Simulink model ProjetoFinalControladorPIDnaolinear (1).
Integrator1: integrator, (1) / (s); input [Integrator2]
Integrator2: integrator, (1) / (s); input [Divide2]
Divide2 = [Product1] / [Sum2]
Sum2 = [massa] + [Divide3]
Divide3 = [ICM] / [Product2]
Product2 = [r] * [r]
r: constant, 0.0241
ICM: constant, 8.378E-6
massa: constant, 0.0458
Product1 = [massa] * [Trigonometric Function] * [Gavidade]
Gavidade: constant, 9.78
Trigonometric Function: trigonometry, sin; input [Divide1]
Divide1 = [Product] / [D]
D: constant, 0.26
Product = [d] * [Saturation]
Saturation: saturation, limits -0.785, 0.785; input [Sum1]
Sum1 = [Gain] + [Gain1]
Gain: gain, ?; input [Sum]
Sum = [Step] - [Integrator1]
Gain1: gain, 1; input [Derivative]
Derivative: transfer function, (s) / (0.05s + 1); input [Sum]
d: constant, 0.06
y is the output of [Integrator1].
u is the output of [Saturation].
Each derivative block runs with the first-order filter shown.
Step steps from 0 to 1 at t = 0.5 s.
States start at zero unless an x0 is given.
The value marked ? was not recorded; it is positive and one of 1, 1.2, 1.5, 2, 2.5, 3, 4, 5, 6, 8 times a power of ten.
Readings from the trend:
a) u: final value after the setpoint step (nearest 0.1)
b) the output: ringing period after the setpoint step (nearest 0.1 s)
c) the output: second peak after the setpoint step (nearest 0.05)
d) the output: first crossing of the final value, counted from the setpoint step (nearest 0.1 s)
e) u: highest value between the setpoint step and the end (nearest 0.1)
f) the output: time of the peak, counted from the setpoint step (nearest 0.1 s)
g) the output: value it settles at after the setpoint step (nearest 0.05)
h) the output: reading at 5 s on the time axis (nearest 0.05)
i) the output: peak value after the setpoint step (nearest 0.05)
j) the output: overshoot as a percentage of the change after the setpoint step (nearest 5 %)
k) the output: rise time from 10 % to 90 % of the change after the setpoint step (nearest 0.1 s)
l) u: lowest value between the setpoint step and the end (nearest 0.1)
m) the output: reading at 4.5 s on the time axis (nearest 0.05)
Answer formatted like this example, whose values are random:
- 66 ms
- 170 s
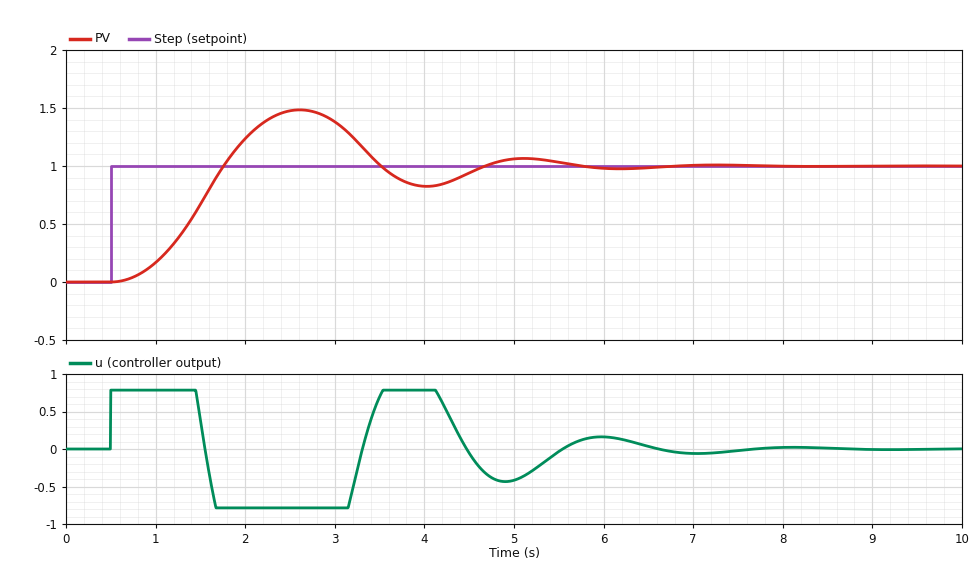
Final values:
- 0.0
- 2.5 s
- 1.05
- 1.3 s
- 0.8
- 2.1 s
- 1.00
- 1.05
- 1.50
- 50 %
- 0.8 s
- -0.8
- 0.95
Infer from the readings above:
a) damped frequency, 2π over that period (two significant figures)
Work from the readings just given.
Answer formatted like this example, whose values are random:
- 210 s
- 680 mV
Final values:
- 2.5 rad/s
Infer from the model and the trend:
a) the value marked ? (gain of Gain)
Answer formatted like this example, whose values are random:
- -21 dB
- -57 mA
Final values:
- 5
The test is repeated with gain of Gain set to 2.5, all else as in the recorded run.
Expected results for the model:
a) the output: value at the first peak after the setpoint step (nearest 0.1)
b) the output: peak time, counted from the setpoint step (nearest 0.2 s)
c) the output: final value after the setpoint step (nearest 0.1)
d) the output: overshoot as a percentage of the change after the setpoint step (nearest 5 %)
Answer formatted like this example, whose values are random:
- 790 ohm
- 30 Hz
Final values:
- 1.2
- 2.0 s
- 1.0
- 20 %
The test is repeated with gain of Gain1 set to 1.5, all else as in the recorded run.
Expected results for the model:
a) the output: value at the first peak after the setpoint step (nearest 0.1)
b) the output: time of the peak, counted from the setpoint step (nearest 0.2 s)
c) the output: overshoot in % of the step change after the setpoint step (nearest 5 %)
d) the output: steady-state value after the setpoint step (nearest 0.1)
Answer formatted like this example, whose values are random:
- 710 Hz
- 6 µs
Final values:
- 1.3
- 2.0 s
- 30 %
- 1.0
